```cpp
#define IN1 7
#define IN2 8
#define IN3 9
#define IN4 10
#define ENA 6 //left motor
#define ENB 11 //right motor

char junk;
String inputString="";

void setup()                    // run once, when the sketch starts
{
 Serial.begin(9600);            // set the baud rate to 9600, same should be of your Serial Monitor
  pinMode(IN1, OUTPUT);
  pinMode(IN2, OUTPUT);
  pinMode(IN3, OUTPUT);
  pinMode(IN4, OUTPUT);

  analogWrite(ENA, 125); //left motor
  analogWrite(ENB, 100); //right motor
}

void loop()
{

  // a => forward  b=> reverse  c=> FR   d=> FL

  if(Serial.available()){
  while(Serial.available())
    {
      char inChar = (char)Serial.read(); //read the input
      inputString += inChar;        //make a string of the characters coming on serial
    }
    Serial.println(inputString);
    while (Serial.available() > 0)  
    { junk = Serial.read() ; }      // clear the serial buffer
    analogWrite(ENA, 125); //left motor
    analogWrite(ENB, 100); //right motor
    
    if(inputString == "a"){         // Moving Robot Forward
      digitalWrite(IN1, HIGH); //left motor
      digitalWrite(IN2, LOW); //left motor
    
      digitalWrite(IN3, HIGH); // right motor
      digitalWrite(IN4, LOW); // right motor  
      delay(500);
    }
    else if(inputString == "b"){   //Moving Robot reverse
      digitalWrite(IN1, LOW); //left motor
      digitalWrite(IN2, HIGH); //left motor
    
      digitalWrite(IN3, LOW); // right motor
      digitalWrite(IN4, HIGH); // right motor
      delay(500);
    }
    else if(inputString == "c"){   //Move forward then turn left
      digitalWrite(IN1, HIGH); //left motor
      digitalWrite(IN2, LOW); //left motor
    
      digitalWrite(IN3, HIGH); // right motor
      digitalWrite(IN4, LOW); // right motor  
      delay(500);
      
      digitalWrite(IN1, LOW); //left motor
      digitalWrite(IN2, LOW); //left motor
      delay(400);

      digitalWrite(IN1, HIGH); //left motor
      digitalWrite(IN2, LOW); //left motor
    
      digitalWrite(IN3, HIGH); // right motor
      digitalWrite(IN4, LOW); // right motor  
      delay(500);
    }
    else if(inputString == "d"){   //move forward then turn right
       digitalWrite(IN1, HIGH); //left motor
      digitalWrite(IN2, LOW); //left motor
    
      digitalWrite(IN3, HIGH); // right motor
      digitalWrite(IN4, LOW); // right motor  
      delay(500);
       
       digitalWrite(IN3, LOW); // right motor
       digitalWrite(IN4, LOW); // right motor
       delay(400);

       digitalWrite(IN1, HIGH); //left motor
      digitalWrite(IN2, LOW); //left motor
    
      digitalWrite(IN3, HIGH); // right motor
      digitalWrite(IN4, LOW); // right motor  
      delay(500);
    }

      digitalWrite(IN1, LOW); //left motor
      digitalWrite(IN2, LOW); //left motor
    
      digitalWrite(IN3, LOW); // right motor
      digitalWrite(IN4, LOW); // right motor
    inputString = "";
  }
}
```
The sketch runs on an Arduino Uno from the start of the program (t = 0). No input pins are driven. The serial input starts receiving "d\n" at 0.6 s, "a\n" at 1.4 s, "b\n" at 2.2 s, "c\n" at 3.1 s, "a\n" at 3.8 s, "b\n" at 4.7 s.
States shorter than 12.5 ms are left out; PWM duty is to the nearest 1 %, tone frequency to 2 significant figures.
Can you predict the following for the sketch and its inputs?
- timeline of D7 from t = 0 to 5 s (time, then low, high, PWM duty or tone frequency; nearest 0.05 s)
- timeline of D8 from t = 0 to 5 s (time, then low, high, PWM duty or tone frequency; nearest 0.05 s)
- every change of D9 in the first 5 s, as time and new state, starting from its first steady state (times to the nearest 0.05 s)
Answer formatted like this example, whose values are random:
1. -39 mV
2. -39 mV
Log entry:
1. 0 s low; 0.6 s high; 2 s low; 3.1 s high; 3.6 s low; 4 s high; 4.5 s low
2. 0 s low; 2.2 s high; 2.7 s low; 4.7 s high
3. 0 s low; 0.6 s high; 1.1 s low; 1.5 s high; 2 s low; 3.1 s high; 4.5 s low
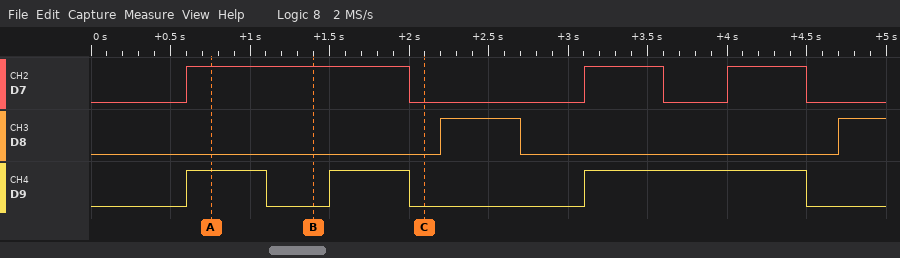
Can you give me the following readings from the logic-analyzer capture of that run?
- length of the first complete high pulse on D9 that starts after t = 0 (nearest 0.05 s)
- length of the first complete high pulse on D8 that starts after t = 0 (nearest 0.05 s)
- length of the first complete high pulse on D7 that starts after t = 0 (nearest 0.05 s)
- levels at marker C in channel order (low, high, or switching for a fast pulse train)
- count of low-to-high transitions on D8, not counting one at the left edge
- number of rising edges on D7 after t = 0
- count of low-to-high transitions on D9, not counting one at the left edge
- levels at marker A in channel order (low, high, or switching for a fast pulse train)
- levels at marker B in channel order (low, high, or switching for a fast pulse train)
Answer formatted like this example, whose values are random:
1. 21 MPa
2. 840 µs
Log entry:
1. 0.50 s
2. 0.50 s
3. 1.40 s
4. D7 low, D8 low, D9 low
5. 2
6. 3
7. 3
8. D7 high, D8 low, D9 high
9. D7 high, D8 low, D9 low
